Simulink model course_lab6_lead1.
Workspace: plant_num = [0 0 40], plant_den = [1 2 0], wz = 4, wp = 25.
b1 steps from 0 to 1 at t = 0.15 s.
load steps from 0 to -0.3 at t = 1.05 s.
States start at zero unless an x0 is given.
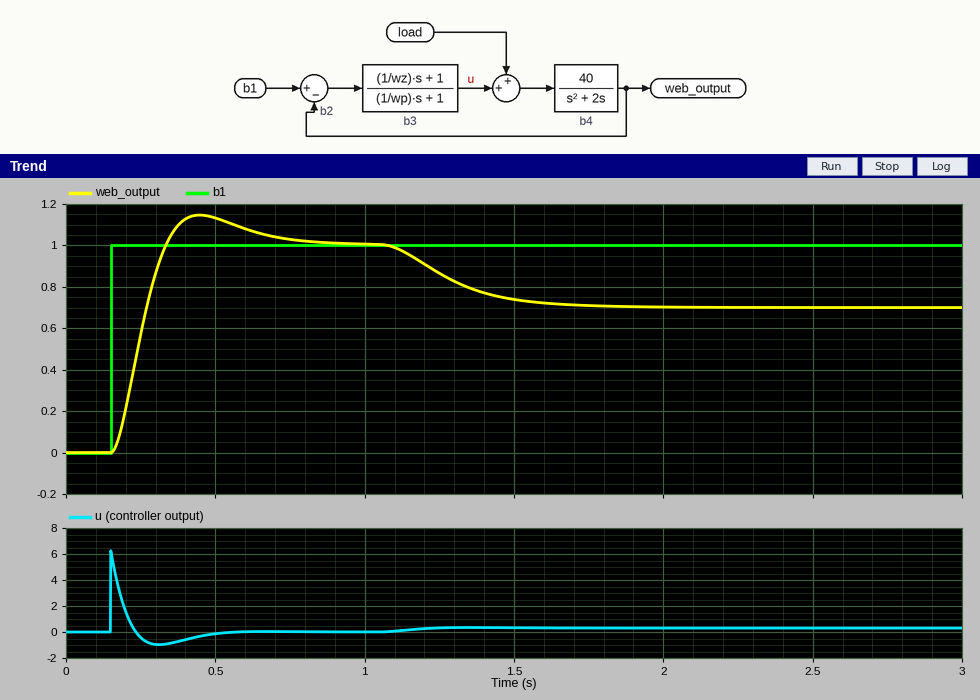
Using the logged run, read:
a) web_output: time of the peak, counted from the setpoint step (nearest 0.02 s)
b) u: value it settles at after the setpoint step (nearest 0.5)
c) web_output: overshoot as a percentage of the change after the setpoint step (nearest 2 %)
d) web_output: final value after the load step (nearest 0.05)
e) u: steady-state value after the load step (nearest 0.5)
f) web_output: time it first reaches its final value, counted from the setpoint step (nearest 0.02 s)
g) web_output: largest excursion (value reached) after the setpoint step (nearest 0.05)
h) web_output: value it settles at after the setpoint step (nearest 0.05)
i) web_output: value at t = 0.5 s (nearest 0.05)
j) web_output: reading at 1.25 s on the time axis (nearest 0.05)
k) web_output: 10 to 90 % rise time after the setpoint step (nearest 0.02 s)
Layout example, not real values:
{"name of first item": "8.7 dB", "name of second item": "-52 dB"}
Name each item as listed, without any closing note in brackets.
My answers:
{"web_output: time of the peak, counted from the setpoint step": "0.30 s", "u: value it settles at after the setpoint step": "0.0", "web_output: overshoot as a percentage of the change after the setpoint step": "14 %", "web_output: final value after the load step": "0.70", "u: steady-state value after the load step": "0.5", "web_output: time it first reaches its final value, counted from the setpoint step": "0.18 s", "web_output: largest excursion (value reached) after the setpoint step": "1.15", "web_output: value it settles at after the setpoint step": "1.00", "web_output: value at t = 0.5 s": "1.15", "web_output: reading at 1.25 s on the time axis": "0.85", "web_output: 10 to 90 % rise time after the setpoint step": "0.12 s"}
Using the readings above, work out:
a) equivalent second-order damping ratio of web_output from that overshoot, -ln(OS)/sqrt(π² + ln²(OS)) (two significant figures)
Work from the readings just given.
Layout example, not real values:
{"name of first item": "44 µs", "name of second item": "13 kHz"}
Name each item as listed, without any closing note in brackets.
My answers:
{"equivalent second-order damping ratio of web_output from that overshoot, -ln(OS)/sqrt(π² + ln²(OS))": "0.53"}
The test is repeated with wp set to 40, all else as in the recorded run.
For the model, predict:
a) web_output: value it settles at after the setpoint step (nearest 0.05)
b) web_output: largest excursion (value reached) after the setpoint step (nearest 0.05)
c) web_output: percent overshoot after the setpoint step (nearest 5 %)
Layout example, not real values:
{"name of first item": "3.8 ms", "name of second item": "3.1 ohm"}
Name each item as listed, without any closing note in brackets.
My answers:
{"web_output: value it settles at after the setpoint step": "1.00", "web_output: largest excursion (value reached) after the setpoint step": "1.10", "web_output: percent overshoot after the setpoint step": "10 %"}
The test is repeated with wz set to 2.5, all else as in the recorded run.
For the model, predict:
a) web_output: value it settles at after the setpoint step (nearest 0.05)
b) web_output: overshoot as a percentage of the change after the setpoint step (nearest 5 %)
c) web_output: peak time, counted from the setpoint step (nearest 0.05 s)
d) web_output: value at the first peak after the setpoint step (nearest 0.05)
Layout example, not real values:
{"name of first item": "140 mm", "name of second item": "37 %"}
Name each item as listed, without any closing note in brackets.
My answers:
{"web_output: value it settles at after the setpoint step": "1.00", "web_output: overshoot as a percentage of the change after the setpoint step": "10 %", "web_output: peak time, counted from the setpoint step": "0.20 s", "web_output: value at the first peak after the setpoint step": "1.10"}
